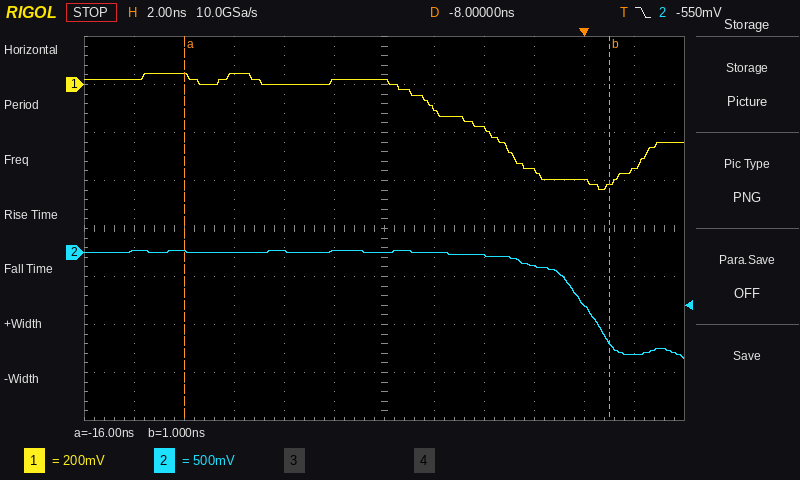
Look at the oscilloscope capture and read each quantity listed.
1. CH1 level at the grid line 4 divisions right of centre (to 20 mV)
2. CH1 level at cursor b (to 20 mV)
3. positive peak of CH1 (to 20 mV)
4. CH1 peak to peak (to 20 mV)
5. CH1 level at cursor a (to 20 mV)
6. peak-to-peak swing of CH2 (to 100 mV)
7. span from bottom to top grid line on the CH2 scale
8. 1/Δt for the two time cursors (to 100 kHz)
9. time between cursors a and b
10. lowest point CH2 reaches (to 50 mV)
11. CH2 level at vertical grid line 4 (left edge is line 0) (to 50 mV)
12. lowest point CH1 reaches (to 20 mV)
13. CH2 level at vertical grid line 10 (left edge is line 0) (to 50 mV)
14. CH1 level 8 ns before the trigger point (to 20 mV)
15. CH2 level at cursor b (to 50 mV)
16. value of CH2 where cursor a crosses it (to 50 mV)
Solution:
-400 mV
-420 mV
40 mV
480 mV
40 mV
1.10 V
4 V
58.8 MHz
17.0 ns
-1.10 V
0 mV
-440 mV
-550 mV
20 mV
-950 mV
0 mV
